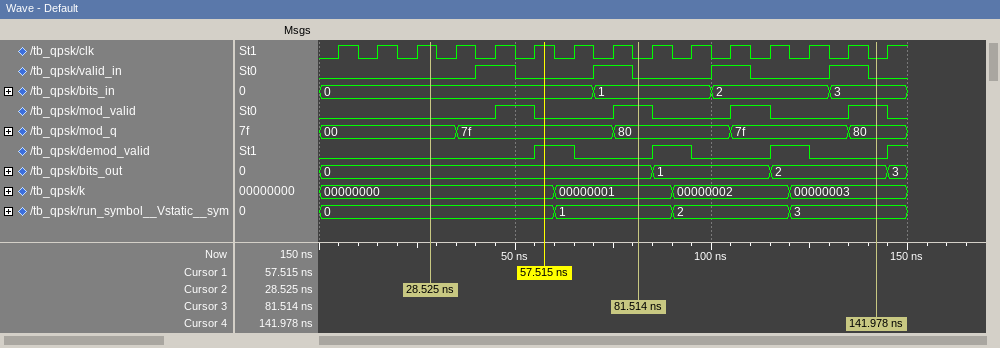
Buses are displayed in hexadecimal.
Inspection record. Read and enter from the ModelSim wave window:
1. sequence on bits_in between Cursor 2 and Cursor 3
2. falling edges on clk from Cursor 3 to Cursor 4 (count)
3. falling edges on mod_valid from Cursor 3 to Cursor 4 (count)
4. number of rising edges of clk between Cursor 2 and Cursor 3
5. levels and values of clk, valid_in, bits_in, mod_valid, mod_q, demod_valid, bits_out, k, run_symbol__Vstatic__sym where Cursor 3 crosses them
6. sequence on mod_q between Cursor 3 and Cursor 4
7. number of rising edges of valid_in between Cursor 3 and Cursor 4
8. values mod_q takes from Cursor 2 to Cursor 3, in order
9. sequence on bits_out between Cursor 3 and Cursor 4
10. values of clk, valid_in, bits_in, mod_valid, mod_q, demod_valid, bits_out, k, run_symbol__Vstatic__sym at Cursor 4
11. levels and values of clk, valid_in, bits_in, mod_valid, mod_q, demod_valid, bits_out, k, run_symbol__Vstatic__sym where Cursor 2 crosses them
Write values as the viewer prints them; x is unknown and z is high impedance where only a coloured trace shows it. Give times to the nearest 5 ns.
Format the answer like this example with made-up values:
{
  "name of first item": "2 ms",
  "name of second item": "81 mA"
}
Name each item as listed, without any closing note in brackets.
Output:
{
  "sequence on bits_in between Cursor 2 and Cursor 3": "0, 1",
  "falling edges on clk from Cursor 3 to Cursor 4": "6",
  "falling edges on mod_valid from Cursor 3 to Cursor 4": "2",
  "number of rising edges of clk between Cursor 2 and Cursor 3": "5",
  "levels and values of clk, valid_in, bits_in, mod_valid, mod_q, demod_valid, bits_out, k, run_symbol__Vstatic__sym where Cursor 3 crosses them": "clk=0, valid_in=0, bits_in=1, mod_valid=1, mod_q=80, demod_valid=0, bits_out=0, k=00000001, run_symbol__Vstatic__sym=1",
  "sequence on mod_q between Cursor 3 and Cursor 4": "80, 7f, 80",
  "number of rising edges of valid_in between Cursor 3 and Cursor 4": "2",
  "values mod_q takes from Cursor 2 to Cursor 3, in order": "00, 7f, 80",
  "sequence on bits_out between Cursor 3 and Cursor 4": "0, 1, 2",
  "values of clk, valid_in, bits_in, mod_valid, mod_q, demod_valid, bits_out, k, run_symbol__Vstatic__sym at Cursor 4": "clk=0, valid_in=0, bits_in=3, mod_valid=1, mod_q=80, demod_valid=0, bits_out=2, k=00000003, run_symbol__Vstatic__sym=3",
  "levels and values of clk, valid_in, bits_in, mod_valid, mod_q, demod_valid, bits_out, k, run_symbol__Vstatic__sym where Cursor 2 crosses them": "clk=1, valid_in=0, bits_in=0, mod_valid=0, mod_q=00, demod_valid=0, bits_out=0, k=00000000, run_symbol__Vstatic__sym=0"
}
